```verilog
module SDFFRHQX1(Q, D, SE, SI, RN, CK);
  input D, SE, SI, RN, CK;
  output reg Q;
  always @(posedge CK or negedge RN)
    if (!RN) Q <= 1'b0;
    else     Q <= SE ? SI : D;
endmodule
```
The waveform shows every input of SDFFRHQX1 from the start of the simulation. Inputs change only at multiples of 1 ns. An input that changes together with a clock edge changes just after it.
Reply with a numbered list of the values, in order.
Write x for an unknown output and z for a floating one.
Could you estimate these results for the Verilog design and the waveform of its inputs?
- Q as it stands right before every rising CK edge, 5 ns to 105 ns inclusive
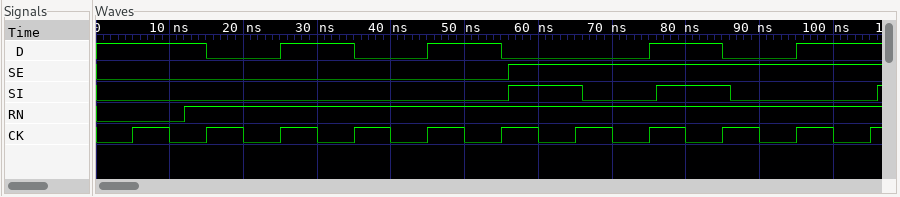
1. 0 0 1 0 1 0 1 1 0 1 0
